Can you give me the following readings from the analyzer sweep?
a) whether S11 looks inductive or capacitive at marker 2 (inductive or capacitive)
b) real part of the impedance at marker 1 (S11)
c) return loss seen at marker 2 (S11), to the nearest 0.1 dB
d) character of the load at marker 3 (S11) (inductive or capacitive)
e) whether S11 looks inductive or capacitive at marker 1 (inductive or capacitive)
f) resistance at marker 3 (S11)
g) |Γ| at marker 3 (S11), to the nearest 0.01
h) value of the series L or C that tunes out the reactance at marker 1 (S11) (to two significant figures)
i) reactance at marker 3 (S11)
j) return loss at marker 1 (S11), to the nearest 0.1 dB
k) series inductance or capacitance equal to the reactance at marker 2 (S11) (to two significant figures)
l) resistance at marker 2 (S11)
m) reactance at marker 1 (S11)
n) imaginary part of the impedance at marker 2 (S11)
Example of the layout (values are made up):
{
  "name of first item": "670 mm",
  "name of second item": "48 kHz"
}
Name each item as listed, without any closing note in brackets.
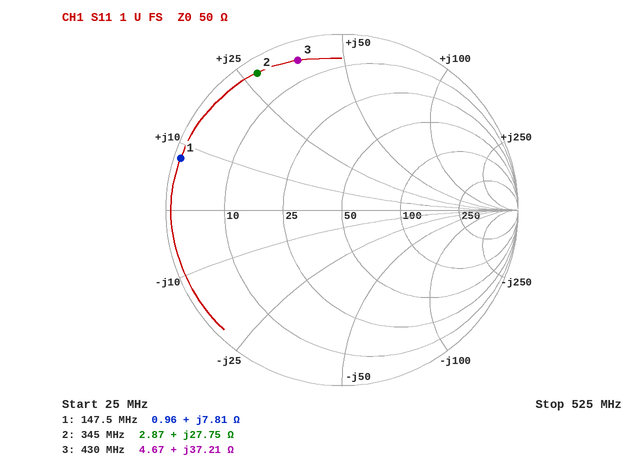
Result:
{
  "whether S11 looks inductive or capacitive at marker 2": "inductive",
  "real part of the impedance at marker 1": "0.96 Ω",
  "return loss seen at marker 2 (S11), to the nearest 0.1 dB": "0.8 dB",
  "character of the load at marker 3 (S11)": "inductive",
  "whether S11 looks inductive or capacitive at marker 1": "inductive",
  "resistance at marker 3": "4.67 Ω",
  "|Γ| at marker 3 (S11), to the nearest 0.01": "0.89",
  "value of the series L or C that tunes out the reactance at marker 1 (S11)": "140 pF",
  "reactance at marker 3": "+37.21 Ω",
  "return loss at marker 1 (S11), to the nearest 0.1 dB": "0.3 dB",
  "series inductance or capacitance equal to the reactance at marker 2 (S11)": "13 nH",
  "resistance at marker 2": "2.87 Ω",
  "reactance at marker 1": "+7.81 Ω",
  "imaginary part of the impedance at marker 2": "+27.75 Ω"
}
